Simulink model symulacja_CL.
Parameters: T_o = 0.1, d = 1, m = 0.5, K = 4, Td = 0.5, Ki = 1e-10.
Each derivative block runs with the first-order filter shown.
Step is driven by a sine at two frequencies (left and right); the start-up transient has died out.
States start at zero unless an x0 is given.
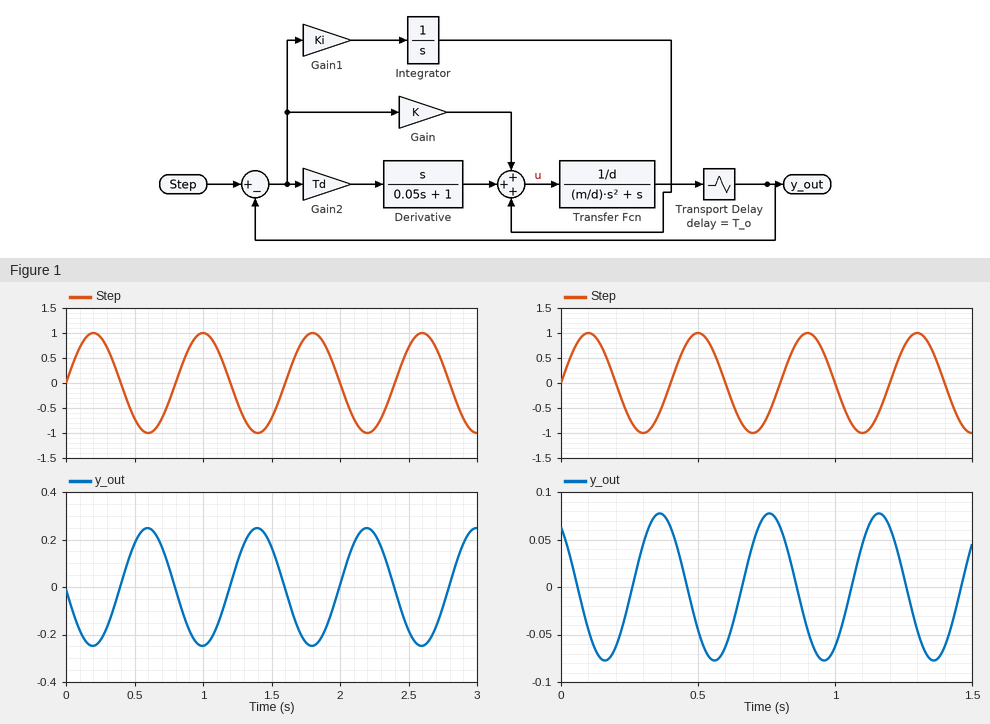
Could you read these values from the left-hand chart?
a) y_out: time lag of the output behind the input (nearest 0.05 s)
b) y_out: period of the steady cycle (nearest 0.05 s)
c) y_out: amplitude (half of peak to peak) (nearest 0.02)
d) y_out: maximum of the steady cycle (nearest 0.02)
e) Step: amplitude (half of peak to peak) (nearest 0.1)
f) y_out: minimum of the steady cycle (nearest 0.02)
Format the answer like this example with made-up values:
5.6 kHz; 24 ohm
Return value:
0.40 s; 0.80 s; 0.24; 0.24; 1.0; -0.24
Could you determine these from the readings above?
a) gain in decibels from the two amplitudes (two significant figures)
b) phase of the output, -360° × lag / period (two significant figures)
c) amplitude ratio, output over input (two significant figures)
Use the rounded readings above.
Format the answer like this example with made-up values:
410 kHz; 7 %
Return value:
-12 dB; -180°; 0.24
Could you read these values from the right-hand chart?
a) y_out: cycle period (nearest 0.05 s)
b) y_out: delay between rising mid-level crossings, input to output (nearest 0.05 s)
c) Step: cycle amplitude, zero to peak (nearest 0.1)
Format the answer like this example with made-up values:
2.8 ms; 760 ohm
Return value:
0.40 s; 0.25 s; 1.0
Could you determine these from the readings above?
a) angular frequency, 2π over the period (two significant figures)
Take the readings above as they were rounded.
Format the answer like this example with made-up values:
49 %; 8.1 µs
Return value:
16 rad/s
